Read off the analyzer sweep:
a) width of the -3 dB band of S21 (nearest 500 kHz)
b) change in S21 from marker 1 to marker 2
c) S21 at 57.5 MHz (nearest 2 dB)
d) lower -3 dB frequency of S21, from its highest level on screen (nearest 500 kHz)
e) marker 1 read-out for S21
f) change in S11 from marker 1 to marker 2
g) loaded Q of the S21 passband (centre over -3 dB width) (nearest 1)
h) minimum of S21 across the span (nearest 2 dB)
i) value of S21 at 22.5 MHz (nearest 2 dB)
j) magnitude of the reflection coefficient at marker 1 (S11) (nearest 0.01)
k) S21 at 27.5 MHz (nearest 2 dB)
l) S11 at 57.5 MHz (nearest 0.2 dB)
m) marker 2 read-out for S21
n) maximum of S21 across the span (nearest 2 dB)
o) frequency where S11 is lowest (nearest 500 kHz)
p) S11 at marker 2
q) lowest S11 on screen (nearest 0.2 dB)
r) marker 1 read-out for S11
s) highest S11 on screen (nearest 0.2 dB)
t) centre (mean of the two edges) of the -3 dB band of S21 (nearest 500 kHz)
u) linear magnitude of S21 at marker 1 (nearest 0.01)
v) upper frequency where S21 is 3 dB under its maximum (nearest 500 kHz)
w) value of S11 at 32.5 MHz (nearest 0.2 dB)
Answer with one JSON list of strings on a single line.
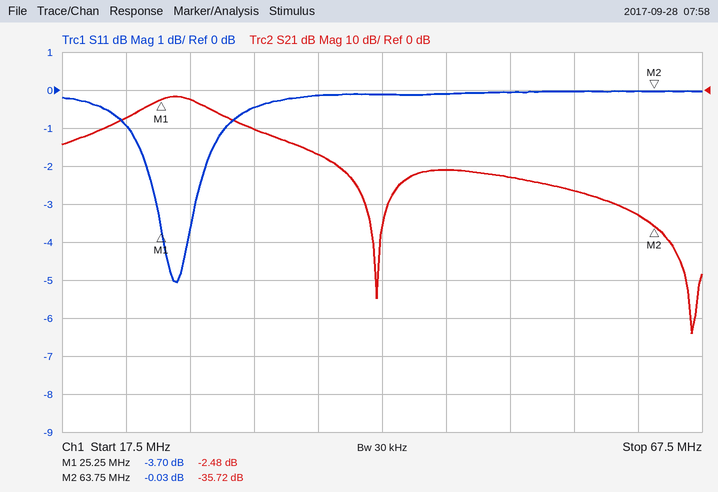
["5.0 MHz", "-33.24 dB", "-26 dB", "24.0 MHz", "-2.48 dB", "3.67 dB", "5", "-64 dB", "-8 dB", "0.65", "-2 dB", "0.0 dB", "-35.72 dB", "-2 dB", "26.5 MHz", "-0.03 dB", "-5.0 dB", "-3.70 dB", "0.0 dB", "26.5 MHz", "0.75", "29.0 MHz", "-0.4 dB"]
